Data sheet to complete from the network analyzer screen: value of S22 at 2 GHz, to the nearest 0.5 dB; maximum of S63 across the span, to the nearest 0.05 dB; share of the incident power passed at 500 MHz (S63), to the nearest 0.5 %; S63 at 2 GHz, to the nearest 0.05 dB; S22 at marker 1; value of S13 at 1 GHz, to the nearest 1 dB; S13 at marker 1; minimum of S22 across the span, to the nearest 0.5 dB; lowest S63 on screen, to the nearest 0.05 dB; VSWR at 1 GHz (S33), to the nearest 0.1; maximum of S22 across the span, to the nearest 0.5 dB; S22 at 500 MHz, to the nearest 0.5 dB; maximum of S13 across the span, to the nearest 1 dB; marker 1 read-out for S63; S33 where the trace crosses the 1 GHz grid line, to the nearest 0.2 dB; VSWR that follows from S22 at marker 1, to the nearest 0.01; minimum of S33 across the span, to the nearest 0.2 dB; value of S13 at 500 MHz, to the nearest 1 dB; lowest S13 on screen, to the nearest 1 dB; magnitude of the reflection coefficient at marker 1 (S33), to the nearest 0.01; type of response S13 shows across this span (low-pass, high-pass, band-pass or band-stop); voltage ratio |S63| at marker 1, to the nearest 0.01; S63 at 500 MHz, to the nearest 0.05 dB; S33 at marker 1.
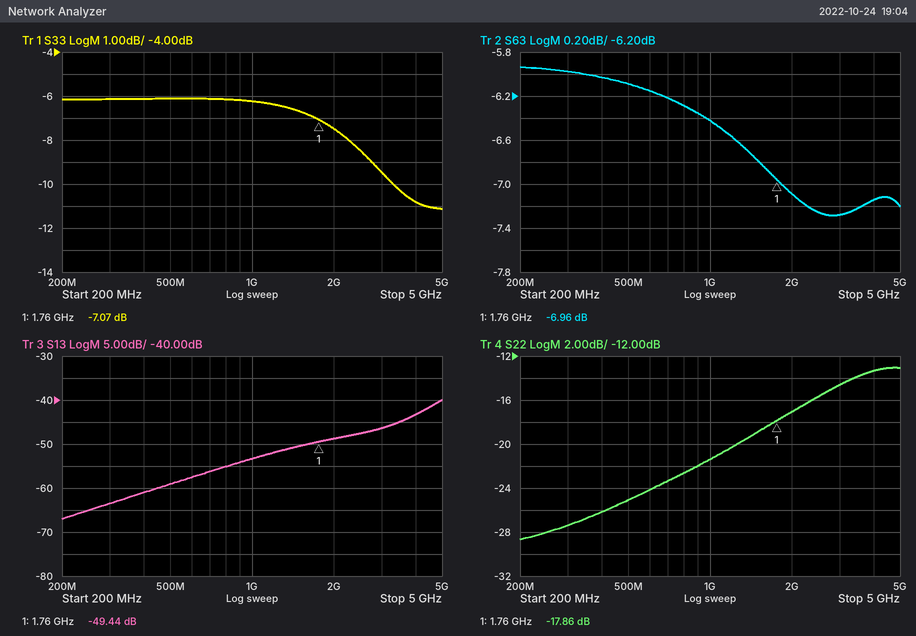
-17.0 dB
-5.95 dB
24.5 %
-7.10 dB
-17.86 dB
-53 dB
-49.44 dB
-28.5 dB
-7.30 dB
2.9
-13.0 dB
-25.0 dB
-40 dB
-6.96 dB
-6.2 dB
1.29
-11.2 dB
-59 dB
-67 dB
0.44
high-pass
0.45
-6.10 dB
-7.07 dB
